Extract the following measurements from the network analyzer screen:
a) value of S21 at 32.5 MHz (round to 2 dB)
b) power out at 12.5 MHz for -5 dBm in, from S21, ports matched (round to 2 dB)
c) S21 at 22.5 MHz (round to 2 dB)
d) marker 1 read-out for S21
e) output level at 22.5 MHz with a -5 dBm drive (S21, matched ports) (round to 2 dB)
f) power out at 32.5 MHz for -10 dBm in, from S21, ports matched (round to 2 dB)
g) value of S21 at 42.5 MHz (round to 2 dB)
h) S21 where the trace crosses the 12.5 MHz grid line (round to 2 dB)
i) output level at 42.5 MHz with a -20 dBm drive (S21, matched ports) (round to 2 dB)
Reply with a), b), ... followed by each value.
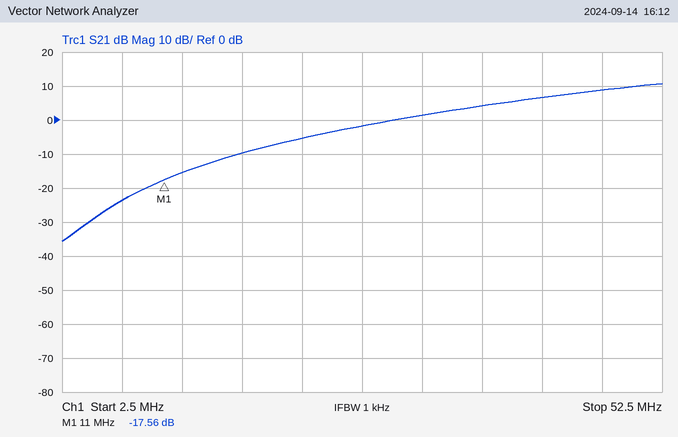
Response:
a) 2 dB
b) -20 dBm
c) -6 dB
d) -17.56 dB
e) -10 dBm
f) -8 dBm
g) 6 dB
h) -16 dB
i) -14 dBm
